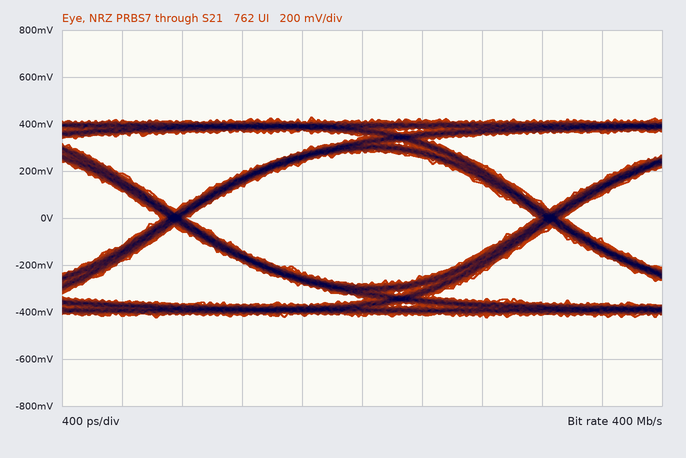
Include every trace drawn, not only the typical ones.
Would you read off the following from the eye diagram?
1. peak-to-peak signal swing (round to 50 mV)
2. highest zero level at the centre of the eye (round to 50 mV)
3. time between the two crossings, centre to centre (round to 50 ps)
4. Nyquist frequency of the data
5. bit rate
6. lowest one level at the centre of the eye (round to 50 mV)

850 mV
-300 mV
2.50 ns
200 MHz
400 Mb/s
300 mV
